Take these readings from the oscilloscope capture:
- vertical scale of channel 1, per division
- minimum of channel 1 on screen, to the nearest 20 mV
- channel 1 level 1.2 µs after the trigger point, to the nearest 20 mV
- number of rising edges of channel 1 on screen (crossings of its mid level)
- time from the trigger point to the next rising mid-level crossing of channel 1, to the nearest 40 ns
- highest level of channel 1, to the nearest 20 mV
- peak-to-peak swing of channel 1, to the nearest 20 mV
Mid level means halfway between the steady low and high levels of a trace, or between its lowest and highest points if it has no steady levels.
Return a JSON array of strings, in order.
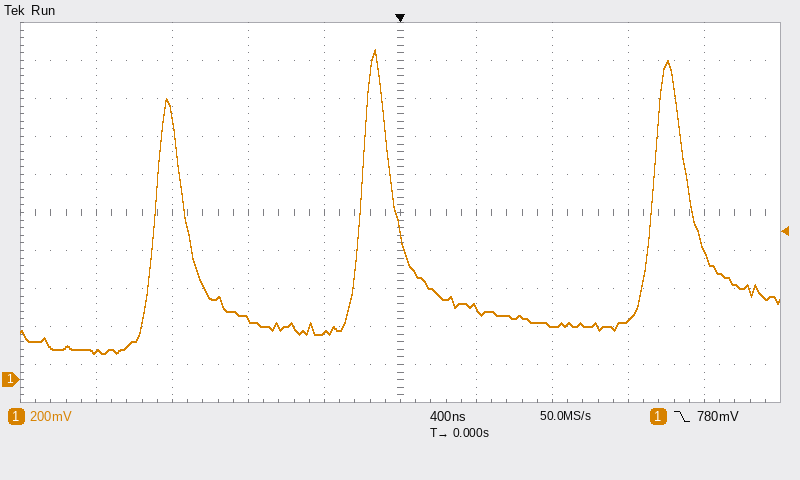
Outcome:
["200 mV", "140 mV", "320 mV", "3", "1.32 µs", "1.74 V", "1.60 V"]
